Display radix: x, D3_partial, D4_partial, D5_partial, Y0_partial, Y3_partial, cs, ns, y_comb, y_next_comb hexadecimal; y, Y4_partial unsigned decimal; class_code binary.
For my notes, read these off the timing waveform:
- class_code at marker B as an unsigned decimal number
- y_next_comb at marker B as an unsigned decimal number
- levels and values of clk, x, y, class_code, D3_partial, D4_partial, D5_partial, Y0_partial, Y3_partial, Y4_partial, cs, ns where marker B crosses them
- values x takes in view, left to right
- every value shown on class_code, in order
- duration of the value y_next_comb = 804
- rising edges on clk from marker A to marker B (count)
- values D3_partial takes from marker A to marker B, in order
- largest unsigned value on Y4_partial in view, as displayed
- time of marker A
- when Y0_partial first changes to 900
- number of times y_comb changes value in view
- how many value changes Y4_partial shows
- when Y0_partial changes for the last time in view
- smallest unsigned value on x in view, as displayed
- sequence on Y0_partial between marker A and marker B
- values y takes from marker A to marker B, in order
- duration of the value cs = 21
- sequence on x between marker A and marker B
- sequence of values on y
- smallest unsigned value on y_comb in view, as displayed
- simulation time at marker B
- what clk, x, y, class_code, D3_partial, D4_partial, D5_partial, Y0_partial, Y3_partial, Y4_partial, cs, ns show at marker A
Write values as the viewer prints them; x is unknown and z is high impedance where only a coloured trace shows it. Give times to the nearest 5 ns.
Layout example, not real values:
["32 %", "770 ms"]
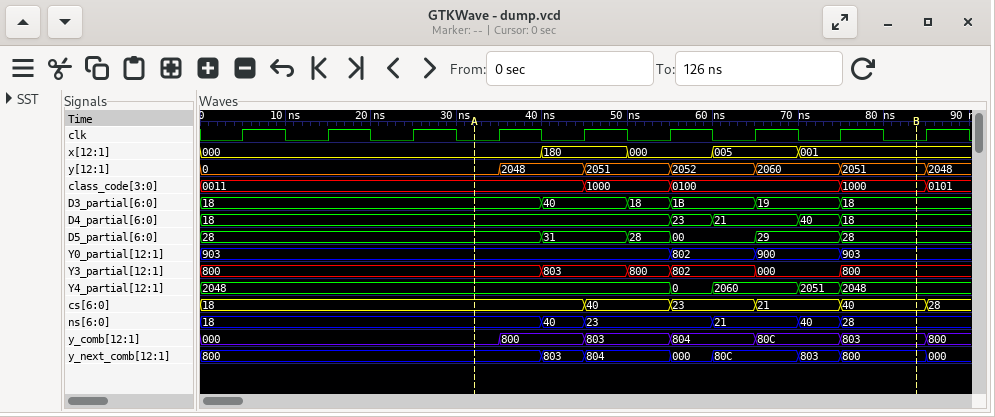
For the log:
["8", "2048", "clk=0, x=001, y=2051, class_code=1000, D3_partial=18, D4_partial=18, D5_partial=28, Y0_partial=903, Y3_partial=800, Y4_partial=2048, cs=40, ns=28", "000, 180, 000, 005, 001", "0011, 1000, 0100, 1000, 0101", "10 ns", "5", "18, 40, 18, 1B, 19, 18", "2060", "30 ns", "65 ns", "6", "4", "75 ns", "000", "903, 802, 900, 903", "0, 2048, 2051, 2052, 2060, 2051", "10 ns", "000, 180, 000, 005, 001", "0, 2048, 2051, 2052, 2060, 2051, 2048", "000", "85 ns", "clk=0, x=000, y=0, class_code=0011, D3_partial=18, D4_partial=18, D5_partial=28, Y0_partial=903, Y3_partial=800, Y4_partial=2048, cs=18, ns=18"]
